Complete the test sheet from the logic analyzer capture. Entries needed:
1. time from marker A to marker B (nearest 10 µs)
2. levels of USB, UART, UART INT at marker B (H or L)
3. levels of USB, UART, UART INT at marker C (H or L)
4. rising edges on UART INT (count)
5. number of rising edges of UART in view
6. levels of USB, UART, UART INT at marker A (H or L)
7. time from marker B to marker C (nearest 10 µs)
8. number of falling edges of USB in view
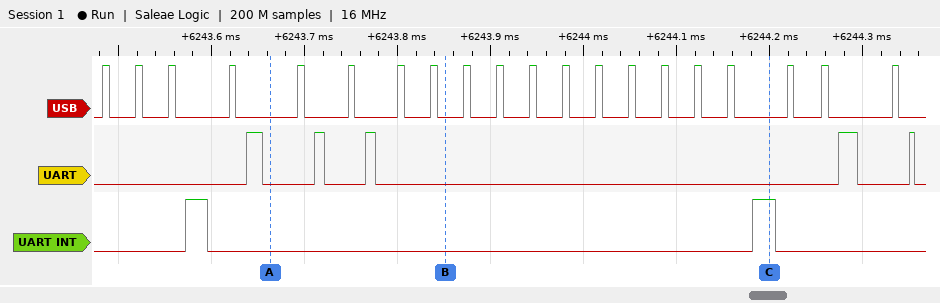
190 µs
USB=L, UART=L, UART INT=L
USB=L, UART=L, UART INT=H
2
5
USB=L, UART=L, UART INT=L
350 µs
20
